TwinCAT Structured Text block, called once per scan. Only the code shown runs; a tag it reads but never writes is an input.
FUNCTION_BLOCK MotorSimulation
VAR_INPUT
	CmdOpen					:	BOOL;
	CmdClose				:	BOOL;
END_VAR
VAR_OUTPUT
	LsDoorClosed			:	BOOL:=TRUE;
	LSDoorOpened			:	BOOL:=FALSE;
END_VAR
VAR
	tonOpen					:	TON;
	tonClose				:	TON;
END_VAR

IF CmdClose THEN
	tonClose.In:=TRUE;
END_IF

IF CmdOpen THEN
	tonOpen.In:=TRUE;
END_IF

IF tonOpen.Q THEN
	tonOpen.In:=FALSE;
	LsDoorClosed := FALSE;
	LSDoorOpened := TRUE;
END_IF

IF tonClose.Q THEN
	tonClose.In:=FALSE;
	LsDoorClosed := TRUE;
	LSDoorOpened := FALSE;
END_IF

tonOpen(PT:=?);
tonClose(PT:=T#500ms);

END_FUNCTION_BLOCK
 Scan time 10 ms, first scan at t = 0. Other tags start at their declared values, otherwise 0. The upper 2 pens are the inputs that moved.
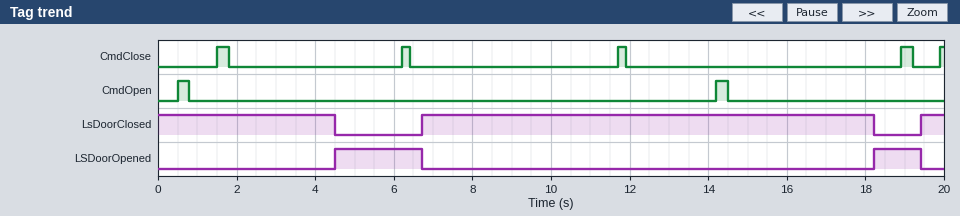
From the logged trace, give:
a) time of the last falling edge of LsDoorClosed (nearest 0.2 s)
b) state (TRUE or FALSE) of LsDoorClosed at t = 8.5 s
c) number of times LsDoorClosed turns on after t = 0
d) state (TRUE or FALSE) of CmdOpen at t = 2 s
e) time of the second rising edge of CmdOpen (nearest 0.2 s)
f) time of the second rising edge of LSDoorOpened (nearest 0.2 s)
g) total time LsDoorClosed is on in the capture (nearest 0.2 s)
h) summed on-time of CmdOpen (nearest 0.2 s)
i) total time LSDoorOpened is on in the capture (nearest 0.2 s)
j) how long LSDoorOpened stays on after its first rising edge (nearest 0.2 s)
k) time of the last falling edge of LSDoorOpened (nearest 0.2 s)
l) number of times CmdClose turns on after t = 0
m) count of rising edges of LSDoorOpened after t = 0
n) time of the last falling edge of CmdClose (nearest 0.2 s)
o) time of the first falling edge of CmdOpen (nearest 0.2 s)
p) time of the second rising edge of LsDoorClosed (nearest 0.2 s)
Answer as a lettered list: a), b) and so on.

a) 18.2 s
b) TRUE
c) 2
d) FALSE
e) 14.2 s
f) 18.2 s
g) 16.6 s
h) 0.6 s
i) 3.4 s
j) 2.2 s
k) 19.4 s
l) 5
m) 2
n) 19.2 s
o) 0.8 s
p) 19.4 s
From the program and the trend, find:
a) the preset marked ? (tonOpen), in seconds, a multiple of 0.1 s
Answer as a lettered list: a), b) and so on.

a) 4.0 s
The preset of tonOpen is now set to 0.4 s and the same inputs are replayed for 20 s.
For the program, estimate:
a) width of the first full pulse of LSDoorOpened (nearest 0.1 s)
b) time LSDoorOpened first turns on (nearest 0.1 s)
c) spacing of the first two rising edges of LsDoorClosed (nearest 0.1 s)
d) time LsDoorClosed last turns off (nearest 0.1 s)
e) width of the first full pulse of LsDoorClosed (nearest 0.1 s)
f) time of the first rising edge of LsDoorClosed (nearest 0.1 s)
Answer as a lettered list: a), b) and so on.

a) 1.1 s
b) 0.9 s
c) 17.4 s
d) 14.6 s
e) 12.6 s
f) 2.0 s
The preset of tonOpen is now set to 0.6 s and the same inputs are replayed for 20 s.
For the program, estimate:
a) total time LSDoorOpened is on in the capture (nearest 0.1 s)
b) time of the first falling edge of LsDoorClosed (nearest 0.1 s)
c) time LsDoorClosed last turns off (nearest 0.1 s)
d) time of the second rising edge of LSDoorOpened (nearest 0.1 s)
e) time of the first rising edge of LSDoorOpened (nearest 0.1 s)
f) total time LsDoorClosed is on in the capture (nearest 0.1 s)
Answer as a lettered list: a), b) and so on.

a) 5.5 s
b) 1.1 s
c) 14.8 s
d) 14.8 s
e) 1.1 s
f) 14.5 s
